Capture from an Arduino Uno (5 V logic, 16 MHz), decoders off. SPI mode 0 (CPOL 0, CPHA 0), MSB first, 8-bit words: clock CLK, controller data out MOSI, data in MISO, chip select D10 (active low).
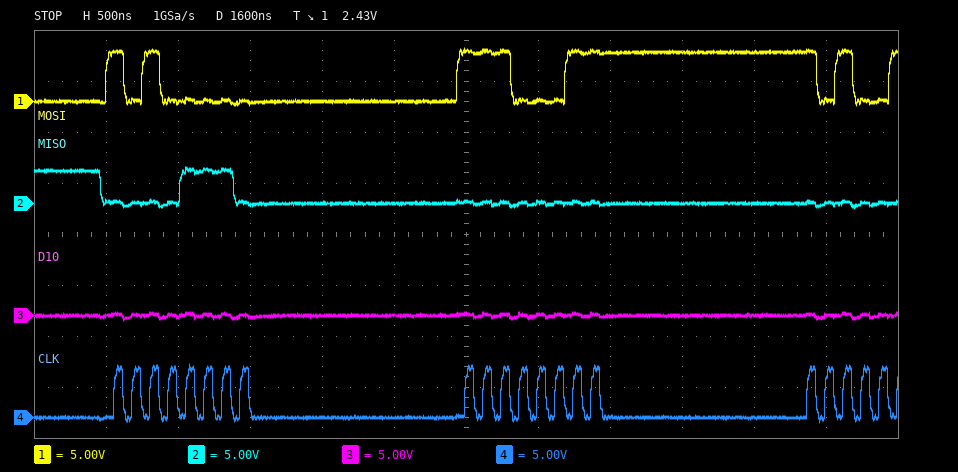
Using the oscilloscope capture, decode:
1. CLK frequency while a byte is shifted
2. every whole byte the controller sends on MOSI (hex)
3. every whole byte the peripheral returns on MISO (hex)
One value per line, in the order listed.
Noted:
8 MHz
0xA0 0xE3
0x0E 0x00
